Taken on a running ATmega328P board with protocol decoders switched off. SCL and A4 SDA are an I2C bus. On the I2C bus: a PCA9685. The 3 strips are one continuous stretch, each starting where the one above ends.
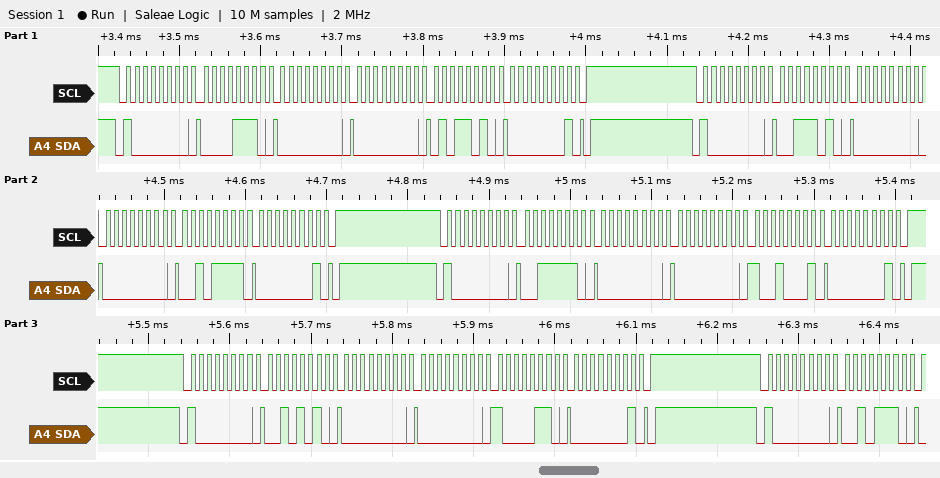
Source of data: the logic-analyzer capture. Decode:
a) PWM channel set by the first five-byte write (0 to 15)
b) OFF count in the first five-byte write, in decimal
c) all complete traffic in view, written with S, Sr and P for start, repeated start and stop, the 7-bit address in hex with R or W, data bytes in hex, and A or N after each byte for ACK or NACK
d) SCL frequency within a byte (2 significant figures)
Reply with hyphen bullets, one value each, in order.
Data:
- 2
- 346
- S 40W A 0E A 00 A 00 A 5A A 01 A P S 40W A 3A A 00 A 00 A 2F A 01 A P S 40W A 3E A 00 A 00 A 91 A 01 A P S 40W A 2A A 00 A 00 A 86 A 01 A P S 40W A 2E A
- 100 kHz
